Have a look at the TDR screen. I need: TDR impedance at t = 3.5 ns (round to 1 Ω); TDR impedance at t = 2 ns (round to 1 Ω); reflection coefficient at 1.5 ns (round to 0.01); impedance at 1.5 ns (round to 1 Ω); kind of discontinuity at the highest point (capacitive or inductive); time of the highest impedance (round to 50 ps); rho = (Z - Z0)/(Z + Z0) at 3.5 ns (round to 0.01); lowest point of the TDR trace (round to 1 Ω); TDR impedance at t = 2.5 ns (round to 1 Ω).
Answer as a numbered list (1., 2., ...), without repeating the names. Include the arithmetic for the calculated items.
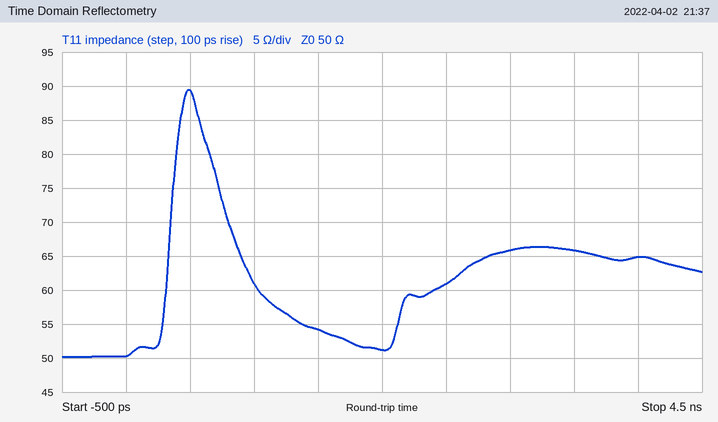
1. 66 Ω
2. 51 Ω
3. (54 − 50)/(54 + 50) ≈ +0.04
4. 54 Ω
5. inductive
6. 500 ps
7. (66 − 50)/(66 + 50) ≈ +0.14
8. 50 Ω
9. 61 Ω
